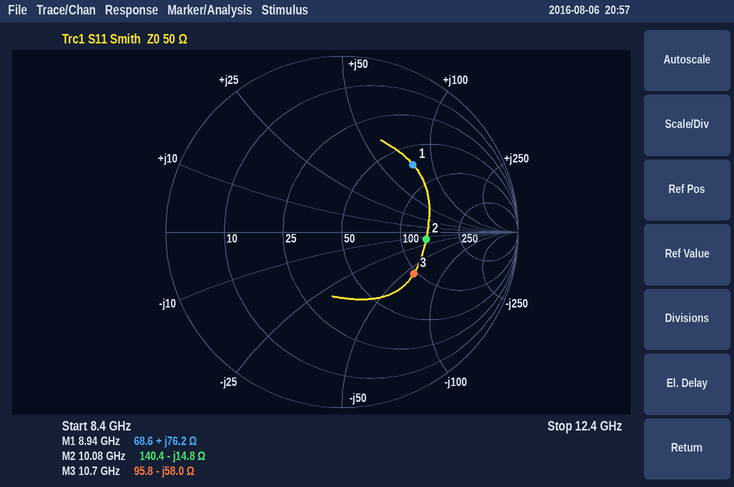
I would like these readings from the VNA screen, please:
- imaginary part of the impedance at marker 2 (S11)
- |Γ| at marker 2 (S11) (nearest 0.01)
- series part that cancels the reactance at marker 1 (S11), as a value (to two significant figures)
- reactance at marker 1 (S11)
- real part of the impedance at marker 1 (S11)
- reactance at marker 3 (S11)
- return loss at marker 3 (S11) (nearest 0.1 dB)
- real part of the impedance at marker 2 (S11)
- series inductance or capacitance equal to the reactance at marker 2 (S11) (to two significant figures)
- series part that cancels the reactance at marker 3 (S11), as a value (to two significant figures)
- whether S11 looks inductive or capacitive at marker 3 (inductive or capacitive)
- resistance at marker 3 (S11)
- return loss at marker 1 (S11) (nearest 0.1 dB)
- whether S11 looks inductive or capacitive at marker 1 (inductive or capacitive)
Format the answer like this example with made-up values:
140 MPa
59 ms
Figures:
-14.8 Ω
0.48
230 fF
+76.2 Ω
68.6 Ω
-58.0 Ω
6.5 dB
140.4 Ω
1.1 pF
860 pH
capacitive
95.8 Ω
5.1 dB
inductive
